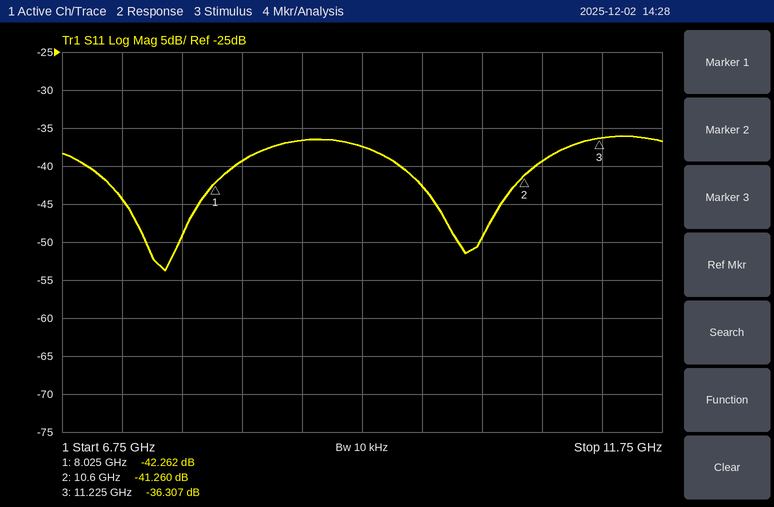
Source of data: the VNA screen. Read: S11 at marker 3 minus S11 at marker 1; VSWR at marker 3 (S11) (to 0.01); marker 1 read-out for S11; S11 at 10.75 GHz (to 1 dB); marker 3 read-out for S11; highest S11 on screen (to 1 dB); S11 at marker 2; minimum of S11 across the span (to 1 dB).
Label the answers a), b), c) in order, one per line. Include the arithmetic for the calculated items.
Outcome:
a) -36.307 − (-42.262) = 5.955 dB
b) (1 + 0.0153)/(1 − 0.0153) ≈ 1.03
c) -42.262 dB
d) -39 dB
e) -36.307 dB
f) -36 dB
g) -41.260 dB
h) -54 dB
